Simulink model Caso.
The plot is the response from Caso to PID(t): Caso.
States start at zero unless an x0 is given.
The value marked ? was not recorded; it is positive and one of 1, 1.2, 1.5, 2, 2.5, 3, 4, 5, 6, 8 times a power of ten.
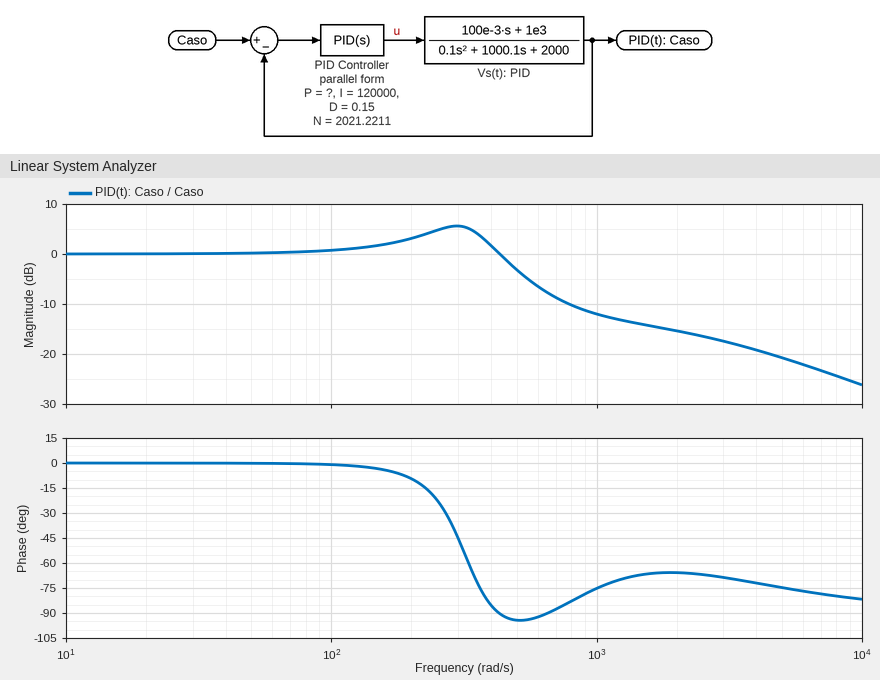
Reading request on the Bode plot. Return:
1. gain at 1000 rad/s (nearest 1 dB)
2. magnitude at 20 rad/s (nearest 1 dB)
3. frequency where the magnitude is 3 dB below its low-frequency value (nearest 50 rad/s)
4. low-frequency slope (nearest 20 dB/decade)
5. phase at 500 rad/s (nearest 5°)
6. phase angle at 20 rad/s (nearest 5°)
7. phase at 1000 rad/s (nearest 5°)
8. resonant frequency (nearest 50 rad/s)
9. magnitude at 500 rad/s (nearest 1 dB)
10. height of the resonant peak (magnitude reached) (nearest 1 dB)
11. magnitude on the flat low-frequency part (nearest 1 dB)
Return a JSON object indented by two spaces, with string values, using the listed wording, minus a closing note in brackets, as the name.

{
  "gain at 1000 rad/s": "-12 dB",
  "magnitude at 20 rad/s": "0 dB",
  "frequency where the magnitude is 3 dB below its low-frequency value": "500 rad/s",
  "low-frequency slope": "0 dB/decade",
  "phase at 500 rad/s": "-95°",
  "phase angle at 20 rad/s": "0°",
  "phase at 1000 rad/s": "-75°",
  "resonant frequency": "300 rad/s",
  "magnitude at 500 rad/s": "-3 dB",
  "height of the resonant peak (magnitude reached)": "6 dB",
  "magnitude on the flat low-frequency part": "0 dB"
}
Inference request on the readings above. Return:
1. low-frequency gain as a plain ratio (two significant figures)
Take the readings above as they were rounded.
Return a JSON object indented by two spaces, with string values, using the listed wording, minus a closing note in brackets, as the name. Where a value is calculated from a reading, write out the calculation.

{
  "low-frequency gain as a plain ratio": "10^(0 / 20) = 1.0"
}
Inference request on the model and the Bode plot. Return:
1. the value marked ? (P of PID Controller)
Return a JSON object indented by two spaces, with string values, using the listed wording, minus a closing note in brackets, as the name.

{
  "the value marked ?": "200"
}
